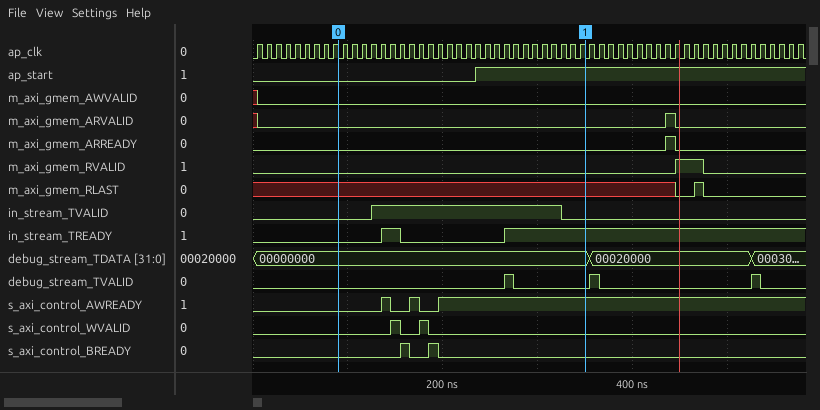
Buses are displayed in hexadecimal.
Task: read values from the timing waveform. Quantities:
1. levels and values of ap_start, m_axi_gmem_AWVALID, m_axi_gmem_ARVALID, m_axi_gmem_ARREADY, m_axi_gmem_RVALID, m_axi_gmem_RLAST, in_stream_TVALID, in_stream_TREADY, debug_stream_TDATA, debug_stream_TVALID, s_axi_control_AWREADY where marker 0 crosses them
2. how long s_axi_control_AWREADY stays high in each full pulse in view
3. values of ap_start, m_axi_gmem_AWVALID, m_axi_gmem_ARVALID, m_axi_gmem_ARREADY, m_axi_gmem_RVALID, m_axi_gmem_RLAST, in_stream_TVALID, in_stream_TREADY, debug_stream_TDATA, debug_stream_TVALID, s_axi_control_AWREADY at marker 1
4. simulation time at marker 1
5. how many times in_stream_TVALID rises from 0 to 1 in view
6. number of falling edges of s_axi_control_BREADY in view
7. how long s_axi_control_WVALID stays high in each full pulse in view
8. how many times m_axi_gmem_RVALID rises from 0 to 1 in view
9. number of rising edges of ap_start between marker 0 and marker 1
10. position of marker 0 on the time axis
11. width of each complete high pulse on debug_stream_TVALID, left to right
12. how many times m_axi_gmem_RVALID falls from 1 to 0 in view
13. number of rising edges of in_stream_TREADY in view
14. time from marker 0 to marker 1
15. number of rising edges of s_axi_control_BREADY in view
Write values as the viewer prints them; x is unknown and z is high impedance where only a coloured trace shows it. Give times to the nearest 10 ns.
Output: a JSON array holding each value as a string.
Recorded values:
["ap_start=0, m_axi_gmem_AWVALID=0, m_axi_gmem_ARVALID=0, m_axi_gmem_ARREADY=0, m_axi_gmem_RVALID=0, m_axi_gmem_RLAST=x, in_stream_TVALID=0, in_stream_TREADY=0, debug_stream_TDATA=00000000, debug_stream_TVALID=0, s_axi_control_AWREADY=0", "10 ns, 10 ns", "ap_start=1, m_axi_gmem_AWVALID=0, m_axi_gmem_ARVALID=0, m_axi_gmem_ARREADY=0, m_axi_gmem_RVALID=0, m_axi_gmem_RLAST=x, in_stream_TVALID=0, in_stream_TREADY=1, debug_stream_TDATA=00000000, debug_stream_TVALID=0, s_axi_control_AWREADY=1", "350 ns", "1", "2", "10 ns, 10 ns", "1", "1", "90 ns", "10 ns, 10 ns, 10 ns", "1", "2", "260 ns", "2"]
